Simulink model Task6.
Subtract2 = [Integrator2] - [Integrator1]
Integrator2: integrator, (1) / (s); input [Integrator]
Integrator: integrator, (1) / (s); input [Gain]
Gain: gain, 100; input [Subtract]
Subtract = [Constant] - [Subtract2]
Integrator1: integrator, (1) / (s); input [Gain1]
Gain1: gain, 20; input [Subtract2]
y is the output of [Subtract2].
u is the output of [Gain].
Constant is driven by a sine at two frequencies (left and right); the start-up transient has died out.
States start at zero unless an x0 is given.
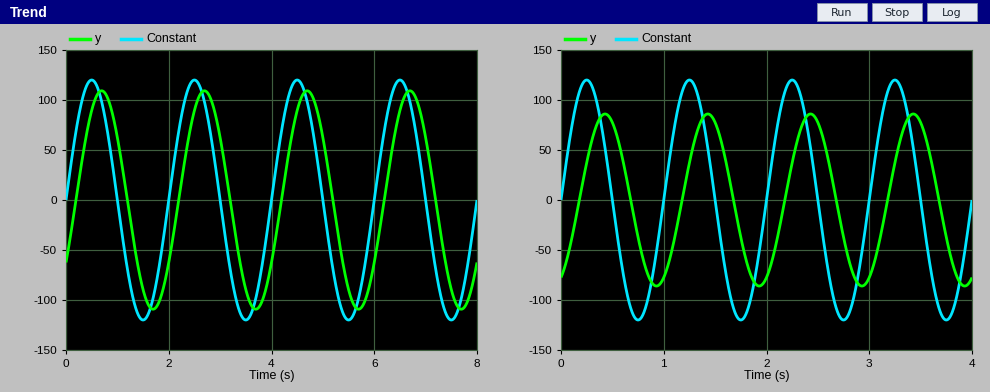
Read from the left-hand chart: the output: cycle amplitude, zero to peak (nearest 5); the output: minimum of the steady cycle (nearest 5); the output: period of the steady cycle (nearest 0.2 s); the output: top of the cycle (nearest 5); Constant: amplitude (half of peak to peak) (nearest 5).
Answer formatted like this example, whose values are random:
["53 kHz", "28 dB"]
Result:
["110", "-110", "2.0 s", "110", "120"]
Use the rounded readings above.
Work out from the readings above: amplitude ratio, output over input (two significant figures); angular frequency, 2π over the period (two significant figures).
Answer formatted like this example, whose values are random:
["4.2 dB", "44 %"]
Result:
["0.92", "3.1 rad/s"]
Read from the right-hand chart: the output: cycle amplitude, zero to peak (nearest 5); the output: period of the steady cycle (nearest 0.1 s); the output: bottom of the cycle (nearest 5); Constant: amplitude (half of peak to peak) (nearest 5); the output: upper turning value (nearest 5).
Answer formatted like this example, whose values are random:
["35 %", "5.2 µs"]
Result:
["85", "1.0 s", "-85", "120", "85"]
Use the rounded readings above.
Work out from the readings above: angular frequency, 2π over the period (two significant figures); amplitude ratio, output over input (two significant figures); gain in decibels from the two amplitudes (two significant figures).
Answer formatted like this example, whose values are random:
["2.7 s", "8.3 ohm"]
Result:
["6.3 rad/s", "0.71", "-3.0 dB"]
